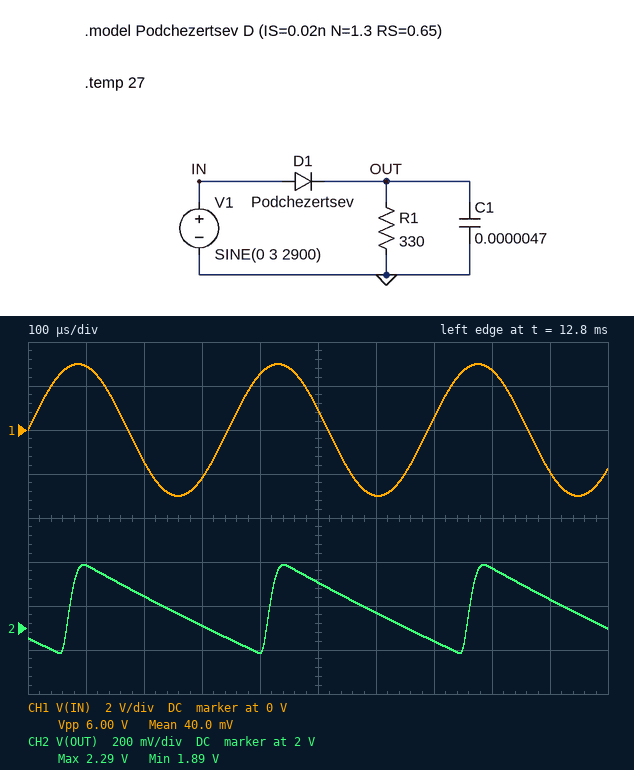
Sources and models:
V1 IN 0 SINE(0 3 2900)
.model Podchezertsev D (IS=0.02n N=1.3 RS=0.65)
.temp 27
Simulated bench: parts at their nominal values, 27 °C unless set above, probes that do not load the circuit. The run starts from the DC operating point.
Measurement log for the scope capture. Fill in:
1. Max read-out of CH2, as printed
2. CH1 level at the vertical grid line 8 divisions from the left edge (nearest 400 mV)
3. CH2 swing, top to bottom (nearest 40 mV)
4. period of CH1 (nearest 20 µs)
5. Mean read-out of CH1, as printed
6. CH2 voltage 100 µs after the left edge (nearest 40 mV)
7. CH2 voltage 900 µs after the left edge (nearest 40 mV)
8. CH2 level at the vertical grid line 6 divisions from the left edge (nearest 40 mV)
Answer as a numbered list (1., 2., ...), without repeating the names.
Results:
1. 2.29 V
2. 2.8 V
3. 400 mV
4. 340 µs
5. 40.0 mV
6. 2.28 V
7. 2.12 V
8. 2.08 V
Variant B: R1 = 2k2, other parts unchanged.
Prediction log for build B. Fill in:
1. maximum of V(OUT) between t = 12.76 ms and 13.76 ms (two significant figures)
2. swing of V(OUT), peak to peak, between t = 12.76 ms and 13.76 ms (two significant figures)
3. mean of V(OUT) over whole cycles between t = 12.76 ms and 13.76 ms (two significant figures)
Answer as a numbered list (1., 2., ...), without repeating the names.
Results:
1. 2.3 V
2. 68 mV
3. 2.3 V
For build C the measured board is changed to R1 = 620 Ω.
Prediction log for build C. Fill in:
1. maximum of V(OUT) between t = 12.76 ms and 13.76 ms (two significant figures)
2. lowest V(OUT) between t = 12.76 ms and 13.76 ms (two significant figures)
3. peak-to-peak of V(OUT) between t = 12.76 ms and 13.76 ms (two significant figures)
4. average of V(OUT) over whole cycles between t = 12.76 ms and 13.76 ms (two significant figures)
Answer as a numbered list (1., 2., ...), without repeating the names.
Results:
1. 2.3 V
2. 2.1 V
3. 230 mV
4. 2.2 V
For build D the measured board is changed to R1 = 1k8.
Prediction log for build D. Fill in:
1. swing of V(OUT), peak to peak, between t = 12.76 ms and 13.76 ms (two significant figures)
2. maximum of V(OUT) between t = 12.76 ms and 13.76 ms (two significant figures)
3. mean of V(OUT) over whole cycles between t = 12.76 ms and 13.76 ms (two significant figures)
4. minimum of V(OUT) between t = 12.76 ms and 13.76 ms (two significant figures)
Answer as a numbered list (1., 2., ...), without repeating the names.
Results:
1. 83 mV
2. 2.3 V
3. 2.3 V
4. 2.2 V
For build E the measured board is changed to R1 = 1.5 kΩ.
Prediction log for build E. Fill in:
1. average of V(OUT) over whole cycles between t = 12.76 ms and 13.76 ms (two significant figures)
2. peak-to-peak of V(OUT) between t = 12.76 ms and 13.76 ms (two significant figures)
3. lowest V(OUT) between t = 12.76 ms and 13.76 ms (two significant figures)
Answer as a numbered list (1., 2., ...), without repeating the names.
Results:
1. 2.3 V
2. 99 mV
3. 2.2 V
